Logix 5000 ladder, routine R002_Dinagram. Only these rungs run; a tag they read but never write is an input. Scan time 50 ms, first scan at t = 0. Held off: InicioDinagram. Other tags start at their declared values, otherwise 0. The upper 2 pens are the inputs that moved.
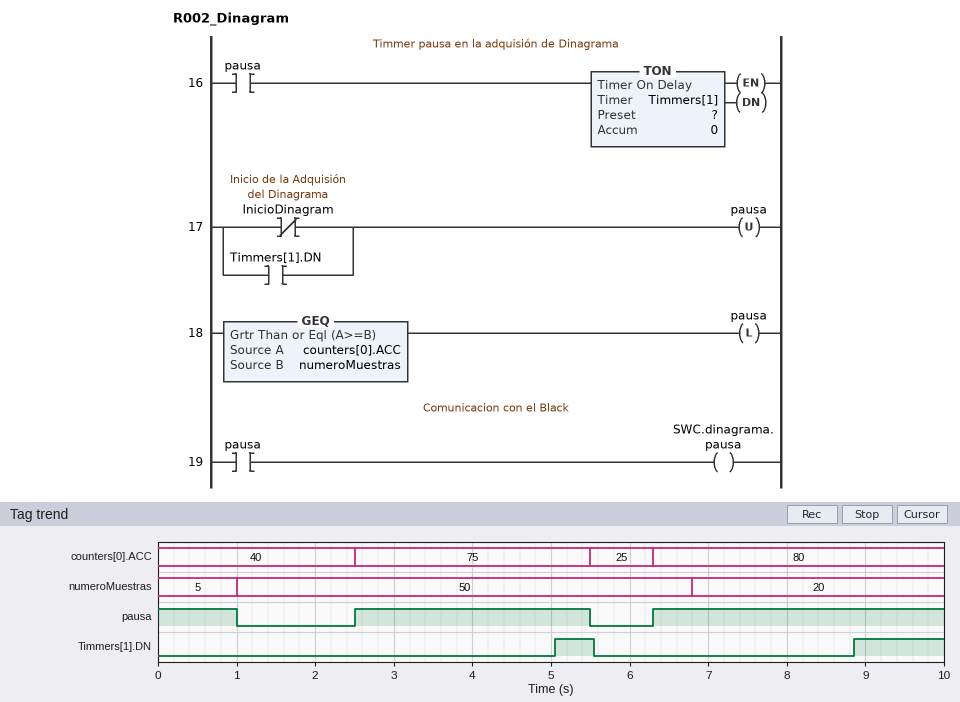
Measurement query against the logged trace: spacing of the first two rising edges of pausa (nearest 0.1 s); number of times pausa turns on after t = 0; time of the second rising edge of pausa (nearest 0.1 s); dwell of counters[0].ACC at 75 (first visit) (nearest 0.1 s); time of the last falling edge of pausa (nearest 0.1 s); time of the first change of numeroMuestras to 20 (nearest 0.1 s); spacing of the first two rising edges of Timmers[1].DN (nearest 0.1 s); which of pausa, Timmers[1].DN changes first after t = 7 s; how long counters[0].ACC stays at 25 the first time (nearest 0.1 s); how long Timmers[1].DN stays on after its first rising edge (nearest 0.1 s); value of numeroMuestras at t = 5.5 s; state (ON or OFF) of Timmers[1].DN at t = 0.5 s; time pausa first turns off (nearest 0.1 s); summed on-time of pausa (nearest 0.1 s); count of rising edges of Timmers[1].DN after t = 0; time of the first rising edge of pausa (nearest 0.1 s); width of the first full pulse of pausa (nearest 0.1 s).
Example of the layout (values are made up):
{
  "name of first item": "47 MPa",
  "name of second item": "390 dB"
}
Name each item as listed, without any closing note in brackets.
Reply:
{
  "spacing of the first two rising edges of pausa": "3.8 s",
  "number of times pausa turns on after t = 0": "2",
  "time of the second rising edge of pausa": "6.3 s",
  "dwell of counters[0].ACC at 75 (first visit)": "3.0 s",
  "time of the last falling edge of pausa": "5.5 s",
  "time of the first change of numeroMuestras to 20": "6.8 s",
  "spacing of the first two rising edges of Timmers[1].DN": "3.8 s",
  "which of pausa, Timmers[1].DN changes first after t = 7 s": "Timmers[1].DN",
  "how long counters[0].ACC stays at 25 the first time": "0.8 s",
  "how long Timmers[1].DN stays on after its first rising edge": "0.5 s",
  "value of numeroMuestras at t = 5.5 s": "50",
  "state (ON or OFF) of Timmers[1].DN at t = 0.5 s": "OFF",
  "time pausa first turns off": "1.0 s",
  "summed on-time of pausa": "7.7 s",
  "count of rising edges of Timmers[1].DN after t = 0": "2",
  "time of the first rising edge of pausa": "2.5 s",
  "width of the first full pulse of pausa": "3.0 s"
}
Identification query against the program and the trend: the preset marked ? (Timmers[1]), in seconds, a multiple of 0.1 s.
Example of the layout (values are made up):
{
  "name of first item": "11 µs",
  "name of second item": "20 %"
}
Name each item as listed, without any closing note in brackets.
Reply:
{
  "the preset marked ? (Timmers[1]), in seconds, a multiple of 0.1 s": "2.5 s"
}
